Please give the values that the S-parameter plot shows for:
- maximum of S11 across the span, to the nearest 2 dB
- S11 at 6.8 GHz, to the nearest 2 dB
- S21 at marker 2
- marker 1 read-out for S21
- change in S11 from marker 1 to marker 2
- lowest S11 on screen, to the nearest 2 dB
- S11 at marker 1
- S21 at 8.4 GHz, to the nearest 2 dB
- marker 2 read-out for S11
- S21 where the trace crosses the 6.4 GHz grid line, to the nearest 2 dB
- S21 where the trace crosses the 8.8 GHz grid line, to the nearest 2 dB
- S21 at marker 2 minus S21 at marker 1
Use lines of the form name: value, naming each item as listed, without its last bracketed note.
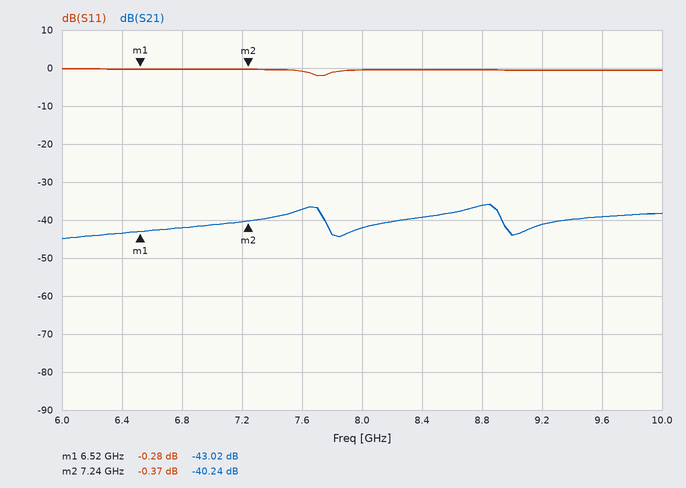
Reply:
maximum of S11 across the span, to the nearest 2 dB: 0 dB
S11 at 6.8 GHz, to the nearest 2 dB: 0 dB
S21 at marker 2: -40.24 dB
marker 1 read-out for S21: -43.02 dB
change in S11 from marker 1 to marker 2: -0.09 dB
lowest S11 on screen, to the nearest 2 dB: -2 dB
S11 at marker 1: -0.28 dB
S21 at 8.4 GHz, to the nearest 2 dB: -40 dB
marker 2 read-out for S11: -0.37 dB
S21 where the trace crosses the 6.4 GHz grid line, to the nearest 2 dB: -44 dB
S21 where the trace crosses the 8.8 GHz grid line, to the nearest 2 dB: -36 dB
S21 at marker 2 minus S21 at marker 1: 2.78 dB
